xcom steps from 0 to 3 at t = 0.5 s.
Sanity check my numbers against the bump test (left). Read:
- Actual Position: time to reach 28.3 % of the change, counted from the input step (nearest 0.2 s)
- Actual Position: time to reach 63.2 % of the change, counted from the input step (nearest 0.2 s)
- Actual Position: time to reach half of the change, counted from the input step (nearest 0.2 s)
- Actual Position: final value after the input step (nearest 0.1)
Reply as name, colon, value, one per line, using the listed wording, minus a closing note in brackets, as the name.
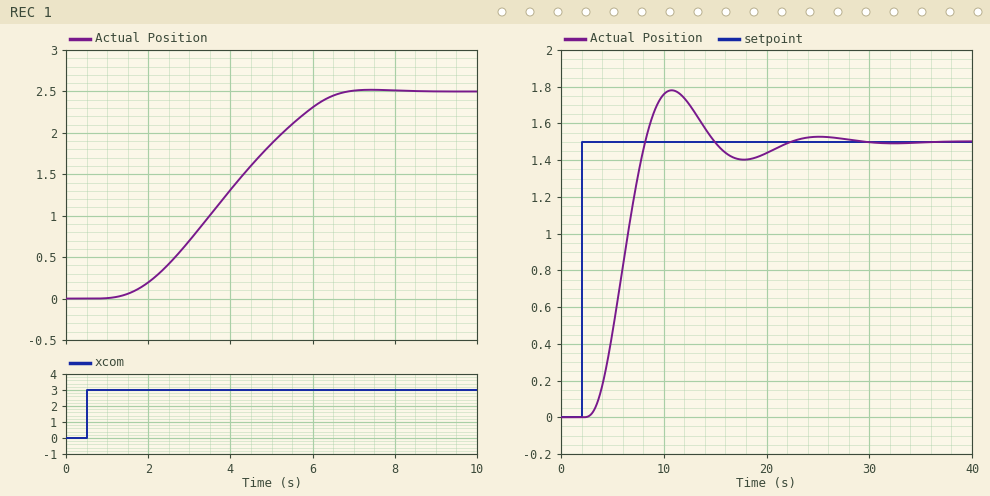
Actual Position: time to reach 28.3 % of the change, counted from the input step: 2.6 s
Actual Position: time to reach 63.2 % of the change, counted from the input step: 4.0 s
Actual Position: time to reach half of the change, counted from the input step: 3.4 s
Actual Position: final value after the input step: 2.5
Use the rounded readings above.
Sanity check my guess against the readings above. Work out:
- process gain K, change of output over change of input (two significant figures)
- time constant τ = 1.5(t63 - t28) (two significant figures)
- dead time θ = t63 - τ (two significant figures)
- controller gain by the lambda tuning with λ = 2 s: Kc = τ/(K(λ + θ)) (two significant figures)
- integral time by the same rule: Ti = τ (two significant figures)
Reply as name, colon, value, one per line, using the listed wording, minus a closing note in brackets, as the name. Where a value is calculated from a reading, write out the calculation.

process gain K, change of output over change of input: (2.5 - 0) / 3 = 0.83
time constant τ = 1.5(t63 - t28): 1.5 × (4 - 2.6) = 2.1 s
dead time θ = t63 - τ: 4 - 2.1 = 1.9 s
controller gain by the lambda tuning with λ = 2 s: Kc = τ/(K(λ + θ)): 2.1 / (0.83 × (2 + 1.9)) = 0.65
integral time by the same rule: Ti = τ: 2.1 s
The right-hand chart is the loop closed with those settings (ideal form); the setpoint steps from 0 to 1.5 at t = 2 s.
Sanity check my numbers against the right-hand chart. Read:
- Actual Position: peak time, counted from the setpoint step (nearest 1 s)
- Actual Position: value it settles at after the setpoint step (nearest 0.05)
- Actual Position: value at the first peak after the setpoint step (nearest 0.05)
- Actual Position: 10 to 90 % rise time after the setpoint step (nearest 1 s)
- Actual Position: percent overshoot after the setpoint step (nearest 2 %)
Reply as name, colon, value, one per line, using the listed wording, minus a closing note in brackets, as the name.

Actual Position: peak time, counted from the setpoint step: 9 s
Actual Position: value it settles at after the setpoint step: 1.50
Actual Position: value at the first peak after the setpoint step: 1.80
Actual Position: 10 to 90 % rise time after the setpoint step: 4 s
Actual Position: percent overshoot after the setpoint step: 18 %
